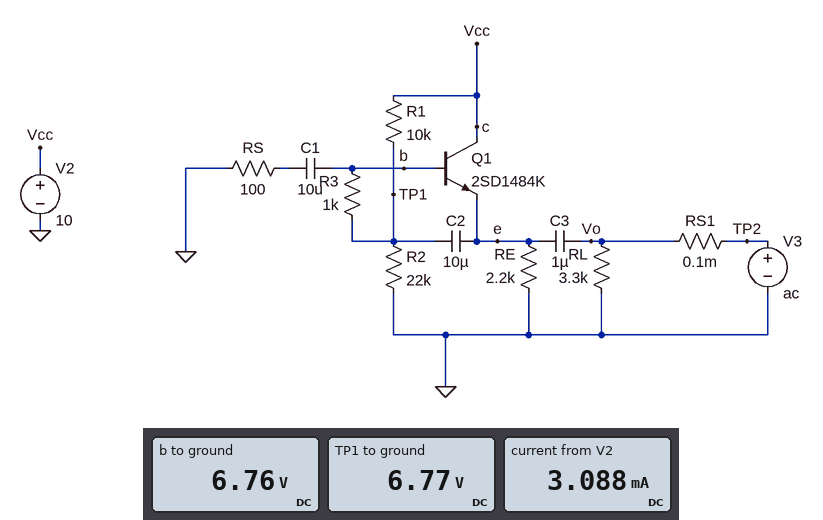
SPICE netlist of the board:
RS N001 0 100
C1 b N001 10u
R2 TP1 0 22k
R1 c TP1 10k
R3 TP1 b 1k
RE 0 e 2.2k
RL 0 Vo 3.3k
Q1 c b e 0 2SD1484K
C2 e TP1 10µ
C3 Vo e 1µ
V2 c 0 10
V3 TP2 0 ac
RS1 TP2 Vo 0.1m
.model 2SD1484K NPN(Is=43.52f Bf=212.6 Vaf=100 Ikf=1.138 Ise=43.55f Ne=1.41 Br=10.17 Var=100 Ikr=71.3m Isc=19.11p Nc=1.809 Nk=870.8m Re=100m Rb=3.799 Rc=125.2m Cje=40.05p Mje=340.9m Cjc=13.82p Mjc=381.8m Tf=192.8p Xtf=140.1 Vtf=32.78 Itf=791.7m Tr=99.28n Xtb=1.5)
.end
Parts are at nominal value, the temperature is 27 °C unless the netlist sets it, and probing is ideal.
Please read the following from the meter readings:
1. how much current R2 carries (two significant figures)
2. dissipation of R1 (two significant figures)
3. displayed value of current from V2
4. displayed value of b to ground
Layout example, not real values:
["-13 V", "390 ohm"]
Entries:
["310 µA", "1.0 mW", "3.088 mA", "6.76 V"]
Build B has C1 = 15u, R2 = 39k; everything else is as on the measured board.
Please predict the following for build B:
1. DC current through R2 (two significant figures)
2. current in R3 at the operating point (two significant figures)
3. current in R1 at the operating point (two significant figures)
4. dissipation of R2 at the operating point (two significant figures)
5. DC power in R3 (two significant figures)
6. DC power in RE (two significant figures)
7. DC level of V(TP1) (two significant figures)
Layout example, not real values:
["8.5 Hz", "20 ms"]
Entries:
["200 µA", "17 µA", "220 µA", "1.6 mW", "300 nW", "23 mW", "7.8 V"]
